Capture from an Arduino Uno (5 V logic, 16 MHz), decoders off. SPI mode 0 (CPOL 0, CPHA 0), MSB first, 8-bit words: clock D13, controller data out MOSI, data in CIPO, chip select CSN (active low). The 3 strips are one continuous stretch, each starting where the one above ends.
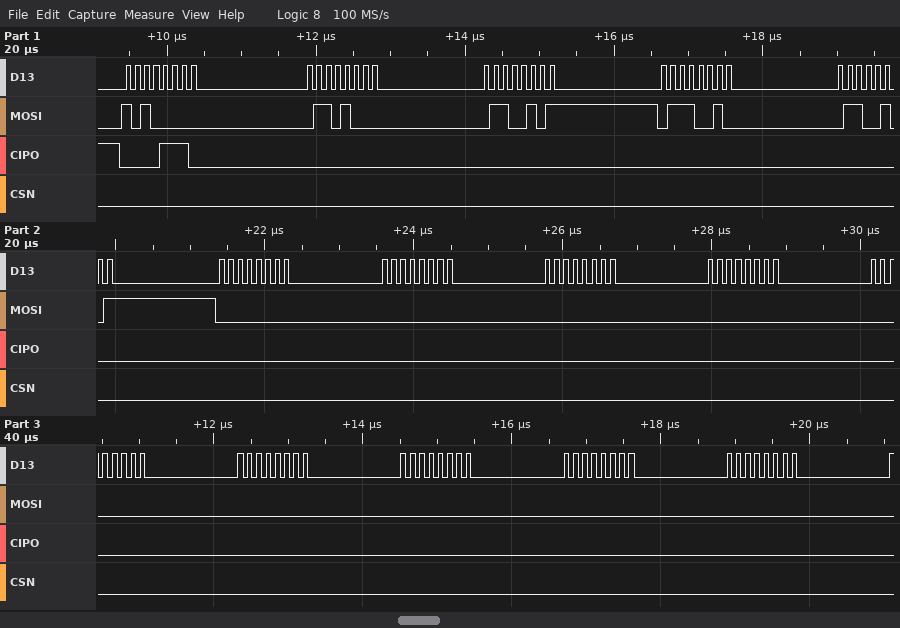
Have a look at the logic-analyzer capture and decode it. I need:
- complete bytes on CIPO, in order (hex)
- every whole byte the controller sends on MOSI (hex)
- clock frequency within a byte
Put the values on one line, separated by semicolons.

0E 00 00 00 00 00 00 00 00 00 00 00 00 00; A0 68 65 72 65 00 00 00 00 00 00 00 00 00; 8 MHz
